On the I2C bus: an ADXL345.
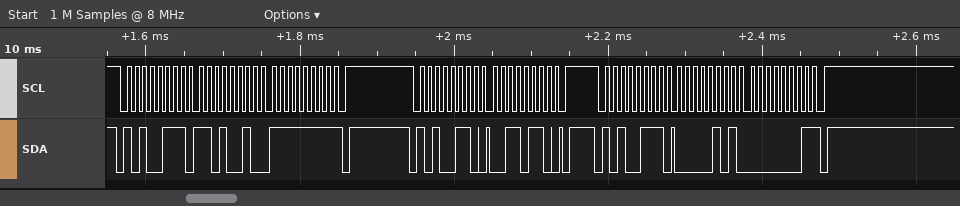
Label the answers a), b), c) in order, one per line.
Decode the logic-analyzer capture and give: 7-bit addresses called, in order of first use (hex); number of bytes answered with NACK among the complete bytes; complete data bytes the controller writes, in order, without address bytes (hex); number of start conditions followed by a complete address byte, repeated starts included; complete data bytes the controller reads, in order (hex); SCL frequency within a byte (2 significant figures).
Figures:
a) 0x53
b) 2
c) 36
d) 3
e) D2 FF 05 01
f) 100 kHz
